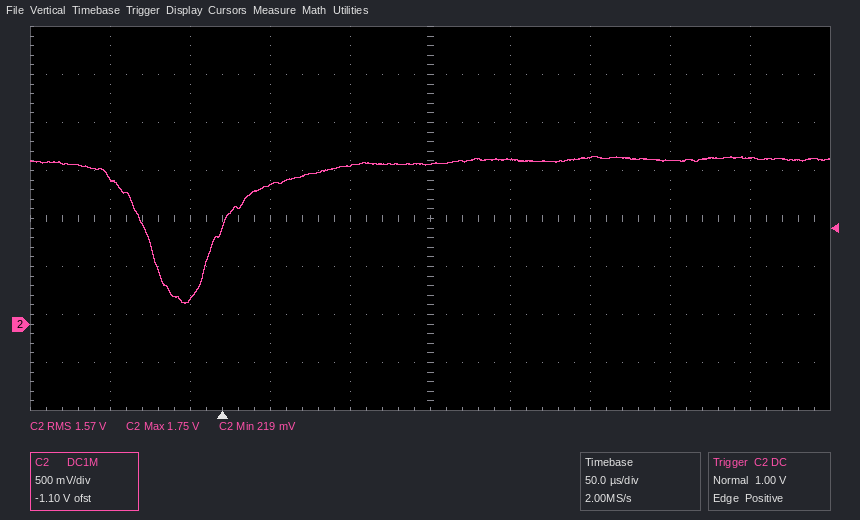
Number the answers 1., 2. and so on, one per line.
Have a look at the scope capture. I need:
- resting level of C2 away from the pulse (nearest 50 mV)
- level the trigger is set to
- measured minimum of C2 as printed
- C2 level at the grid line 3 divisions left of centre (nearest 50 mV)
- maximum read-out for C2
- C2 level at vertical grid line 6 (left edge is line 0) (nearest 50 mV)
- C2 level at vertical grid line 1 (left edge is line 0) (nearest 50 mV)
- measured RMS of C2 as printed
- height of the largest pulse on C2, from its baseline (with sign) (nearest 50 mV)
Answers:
1. 1.70 V
2. 1.00 V
3. 219 mV
4. 250 mV
5. 1.75 V
6. 1.70 V
7. 1.55 V
8. 1.57 V
9. -1.50 V
